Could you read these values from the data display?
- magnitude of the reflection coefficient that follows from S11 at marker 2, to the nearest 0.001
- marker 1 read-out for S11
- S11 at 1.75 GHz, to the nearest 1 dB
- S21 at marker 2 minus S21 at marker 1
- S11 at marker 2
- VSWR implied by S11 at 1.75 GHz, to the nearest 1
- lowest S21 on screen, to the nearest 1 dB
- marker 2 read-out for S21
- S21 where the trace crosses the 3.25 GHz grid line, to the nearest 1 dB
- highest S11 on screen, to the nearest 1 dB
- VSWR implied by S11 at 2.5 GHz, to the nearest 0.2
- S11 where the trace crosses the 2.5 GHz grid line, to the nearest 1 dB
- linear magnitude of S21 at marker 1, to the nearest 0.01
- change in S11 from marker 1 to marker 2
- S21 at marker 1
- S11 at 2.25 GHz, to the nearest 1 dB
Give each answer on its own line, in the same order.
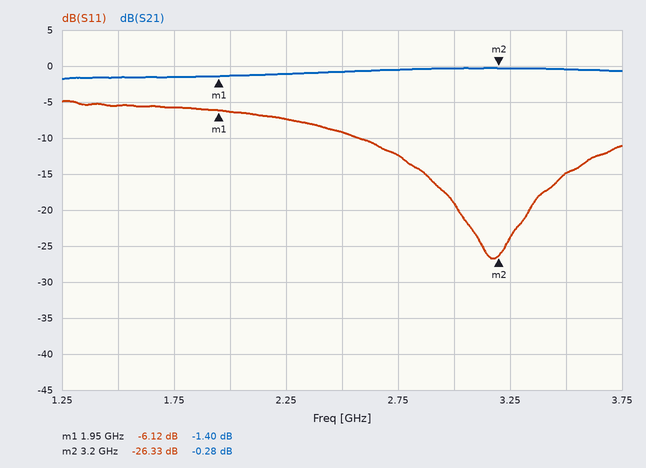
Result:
0.048
-6.12 dB
-6 dB
1.12 dB
-26.33 dB
3
-2 dB
-0.28 dB
0 dB
-5 dB
2.0
-9 dB
0.85
-20.21 dB
-1.40 dB
-7 dB
